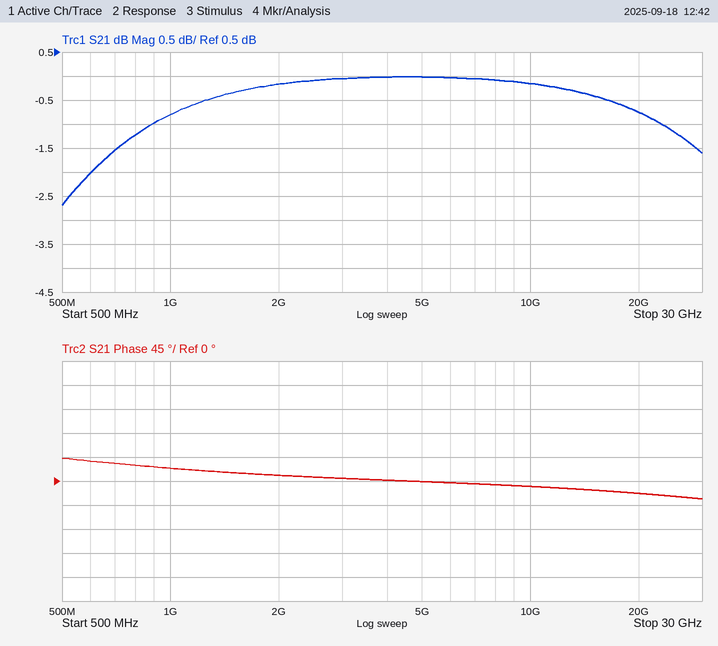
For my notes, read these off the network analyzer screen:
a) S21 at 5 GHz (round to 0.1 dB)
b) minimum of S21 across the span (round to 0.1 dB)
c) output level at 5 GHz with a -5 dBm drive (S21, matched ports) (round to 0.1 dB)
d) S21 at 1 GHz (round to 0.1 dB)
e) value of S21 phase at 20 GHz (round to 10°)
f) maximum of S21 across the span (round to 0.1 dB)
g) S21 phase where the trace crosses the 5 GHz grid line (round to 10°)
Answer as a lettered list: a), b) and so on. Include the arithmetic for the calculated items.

a) 0.0 dB
b) -2.7 dB
c) -5 dBm + (0.0 dB) = -5.0 dBm
d) -0.8 dB
e) -20°
f) 0.0 dB
g) 0°
